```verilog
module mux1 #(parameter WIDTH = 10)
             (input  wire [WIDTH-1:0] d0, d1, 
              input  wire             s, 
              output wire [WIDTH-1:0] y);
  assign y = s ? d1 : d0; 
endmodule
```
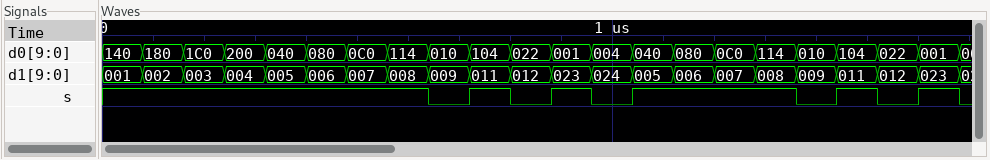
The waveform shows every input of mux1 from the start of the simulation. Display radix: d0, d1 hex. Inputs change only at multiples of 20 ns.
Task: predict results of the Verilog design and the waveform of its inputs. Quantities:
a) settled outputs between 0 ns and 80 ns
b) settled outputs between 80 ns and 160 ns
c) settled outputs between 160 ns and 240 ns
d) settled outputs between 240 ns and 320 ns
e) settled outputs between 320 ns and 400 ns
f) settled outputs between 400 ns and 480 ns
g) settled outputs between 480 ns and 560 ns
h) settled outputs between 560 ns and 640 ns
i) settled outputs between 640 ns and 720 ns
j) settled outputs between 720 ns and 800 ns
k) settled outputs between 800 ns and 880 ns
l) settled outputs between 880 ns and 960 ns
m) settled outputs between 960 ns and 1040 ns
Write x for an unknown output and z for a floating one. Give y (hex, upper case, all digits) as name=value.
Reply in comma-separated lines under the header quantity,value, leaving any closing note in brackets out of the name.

quantity,value
settled outputs between 0 ns and 80 ns,y=001
settled outputs between 80 ns and 160 ns,y=002
settled outputs between 160 ns and 240 ns,y=003
settled outputs between 240 ns and 320 ns,y=004
settled outputs between 320 ns and 400 ns,y=005
settled outputs between 400 ns and 480 ns,y=006
settled outputs between 480 ns and 560 ns,y=007
settled outputs between 560 ns and 640 ns,y=008
settled outputs between 640 ns and 720 ns,y=010
settled outputs between 720 ns and 800 ns,y=011
settled outputs between 800 ns and 880 ns,y=022
settled outputs between 880 ns and 960 ns,y=023
settled outputs between 960 ns and 1040 ns,y=004
